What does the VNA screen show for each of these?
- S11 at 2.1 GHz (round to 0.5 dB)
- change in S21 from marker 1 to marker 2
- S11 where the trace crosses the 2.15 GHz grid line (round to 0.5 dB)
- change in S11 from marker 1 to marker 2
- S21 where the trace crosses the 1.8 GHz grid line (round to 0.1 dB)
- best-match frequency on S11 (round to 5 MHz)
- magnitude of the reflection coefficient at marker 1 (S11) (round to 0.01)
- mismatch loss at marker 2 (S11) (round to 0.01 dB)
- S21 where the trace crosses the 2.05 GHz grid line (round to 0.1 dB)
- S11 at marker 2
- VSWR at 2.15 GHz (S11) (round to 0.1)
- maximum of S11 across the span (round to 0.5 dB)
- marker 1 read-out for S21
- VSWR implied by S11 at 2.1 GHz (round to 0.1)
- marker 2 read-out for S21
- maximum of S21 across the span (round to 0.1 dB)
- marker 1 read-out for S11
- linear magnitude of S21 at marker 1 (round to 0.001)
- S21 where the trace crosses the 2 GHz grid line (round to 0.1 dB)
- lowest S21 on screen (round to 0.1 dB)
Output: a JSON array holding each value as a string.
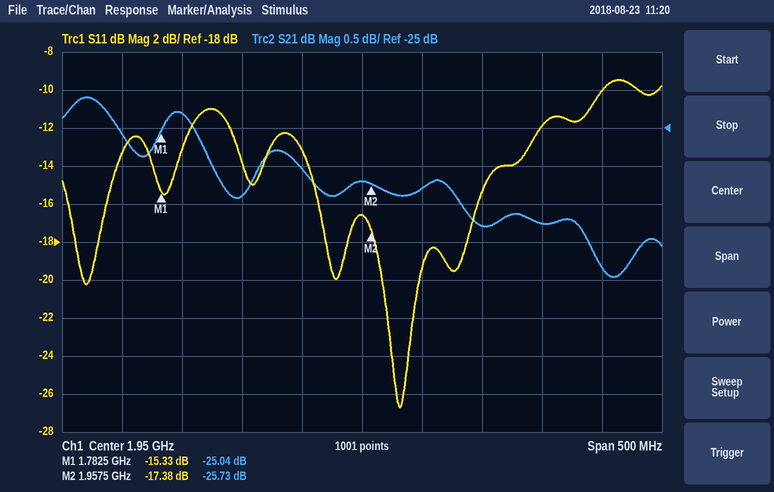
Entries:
["-12.0 dB", "-0.69 dB", "-10.0 dB", "-2.05 dB", "-24.8 dB", "1.980 GHz", "0.17", "0.08 dB", "-26.3 dB", "-17.38 dB", "1.9", "-9.5 dB", "-25.04 dB", "1.7", "-25.73 dB", "-24.6 dB", "-15.33 dB", "0.056", "-25.8 dB", "-27.0 dB"]
